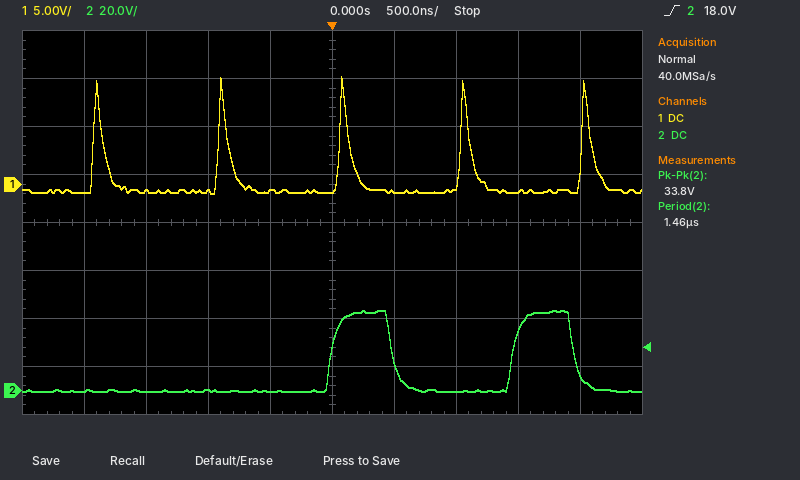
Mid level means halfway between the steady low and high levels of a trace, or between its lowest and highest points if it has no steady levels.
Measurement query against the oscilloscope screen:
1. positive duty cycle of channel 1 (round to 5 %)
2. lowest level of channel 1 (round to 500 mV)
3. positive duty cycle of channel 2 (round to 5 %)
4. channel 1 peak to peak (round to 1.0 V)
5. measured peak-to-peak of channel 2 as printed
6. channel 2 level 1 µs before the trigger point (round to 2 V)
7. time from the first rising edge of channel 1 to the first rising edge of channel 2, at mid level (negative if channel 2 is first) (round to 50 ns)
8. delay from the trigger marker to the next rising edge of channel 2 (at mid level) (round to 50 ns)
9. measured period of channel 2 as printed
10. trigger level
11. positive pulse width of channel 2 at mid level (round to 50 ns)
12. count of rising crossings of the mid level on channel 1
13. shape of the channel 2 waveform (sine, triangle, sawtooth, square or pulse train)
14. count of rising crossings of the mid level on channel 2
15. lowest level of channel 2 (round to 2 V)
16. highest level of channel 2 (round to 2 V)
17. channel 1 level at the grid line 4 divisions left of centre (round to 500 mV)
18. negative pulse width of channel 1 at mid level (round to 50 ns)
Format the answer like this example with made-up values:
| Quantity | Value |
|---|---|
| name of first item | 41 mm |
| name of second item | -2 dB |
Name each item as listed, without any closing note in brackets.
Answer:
| Quantity | Value |
|---|---|
| positive duty cycle of channel 1 | 5 % |
| lowest level of channel 1 | -1.0 V |
| positive duty cycle of channel 2 | 35 % |
| channel 1 peak to peak | 12.0 V |
| measured peak-to-peak of channel 2 as printed | 33.8 V |
| channel 2 level 1 µs before the trigger point | 0 V |
| time from the first rising edge of channel 1 to the first rising edge of channel 2, at mid level (negative if channel 2 is first) | +1.90 µs |
| delay from the trigger marker to the next rising edge of channel 2 (at mid level) | 1.45 µs |
| measured period of channel 2 as printed | 1.46 µs |
| trigger level | 18.0 V |
| positive pulse width of channel 2 at mid level | 500 ns |
| count of rising crossings of the mid level on channel 1 | 5 |
| shape of the channel 2 waveform | pulse train |
| count of rising crossings of the mid level on channel 2 | 2 |
| lowest level of channel 2 | 0 V |
| highest level of channel 2 | 34 V |
| channel 1 level at the grid line 4 divisions left of centre | -1.0 V |
| negative pulse width of channel 1 at mid level | 900 ns |
